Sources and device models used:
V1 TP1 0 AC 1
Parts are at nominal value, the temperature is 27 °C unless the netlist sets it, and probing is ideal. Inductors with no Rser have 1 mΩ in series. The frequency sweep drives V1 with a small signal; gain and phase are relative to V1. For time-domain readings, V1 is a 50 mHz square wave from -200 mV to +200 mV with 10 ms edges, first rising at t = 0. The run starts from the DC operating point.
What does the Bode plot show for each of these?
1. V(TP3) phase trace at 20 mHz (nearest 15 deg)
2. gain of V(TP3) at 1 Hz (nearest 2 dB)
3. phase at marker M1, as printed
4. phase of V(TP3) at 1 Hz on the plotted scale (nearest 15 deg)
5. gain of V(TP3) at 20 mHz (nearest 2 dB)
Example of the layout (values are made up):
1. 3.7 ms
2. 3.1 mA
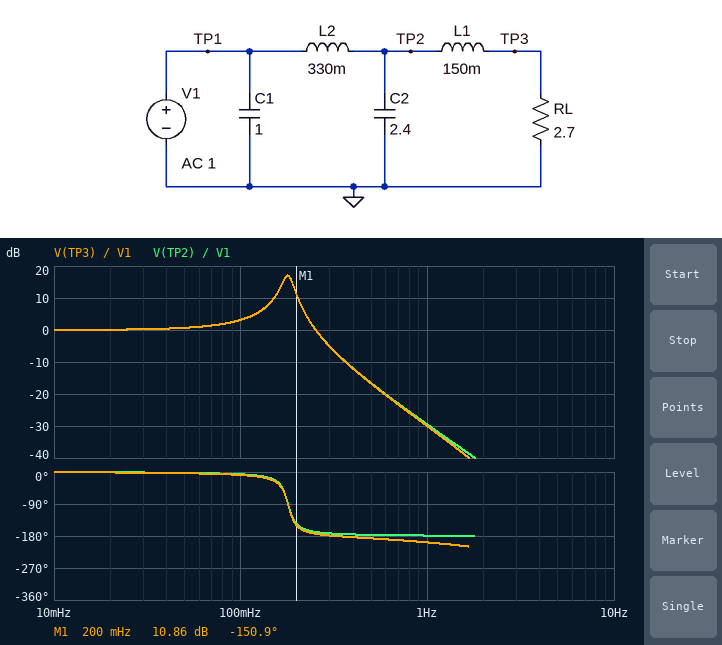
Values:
1. 0 deg
2. -30 dB
3. -150.9 deg
4. -195 deg
5. 0 dB
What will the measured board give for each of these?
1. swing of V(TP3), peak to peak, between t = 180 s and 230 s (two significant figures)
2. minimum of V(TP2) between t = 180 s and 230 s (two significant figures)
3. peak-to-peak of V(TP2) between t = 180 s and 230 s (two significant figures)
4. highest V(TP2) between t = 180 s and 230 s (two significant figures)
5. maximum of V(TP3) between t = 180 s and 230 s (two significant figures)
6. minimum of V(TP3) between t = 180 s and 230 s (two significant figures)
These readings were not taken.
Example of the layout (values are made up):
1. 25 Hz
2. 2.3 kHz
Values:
1. 950 mV
2. -470 mV
3. 950 mV
4. 470 mV
5. 470 mV
6. -470 mV
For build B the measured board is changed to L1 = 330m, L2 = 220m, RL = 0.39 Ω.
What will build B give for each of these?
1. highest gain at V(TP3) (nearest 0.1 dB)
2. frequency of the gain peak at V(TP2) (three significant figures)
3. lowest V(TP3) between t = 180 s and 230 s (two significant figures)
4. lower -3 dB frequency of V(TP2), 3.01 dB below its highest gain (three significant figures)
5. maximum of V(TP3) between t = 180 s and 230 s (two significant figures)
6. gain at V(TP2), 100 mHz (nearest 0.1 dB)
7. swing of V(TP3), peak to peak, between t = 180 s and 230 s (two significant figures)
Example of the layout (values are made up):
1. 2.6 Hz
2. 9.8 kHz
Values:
1. 5.2 dB
2. 264 mHz
3. -270 mV
4. 229 mHz
5. 270 mV
6. 0.2 dB
7. 530 mV
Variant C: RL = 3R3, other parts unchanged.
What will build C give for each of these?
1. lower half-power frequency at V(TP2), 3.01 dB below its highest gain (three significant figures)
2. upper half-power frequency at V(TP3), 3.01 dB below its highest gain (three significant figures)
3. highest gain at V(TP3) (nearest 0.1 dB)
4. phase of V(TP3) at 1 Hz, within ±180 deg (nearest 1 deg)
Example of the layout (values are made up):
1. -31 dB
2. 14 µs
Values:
1. 168 mHz
2. 189 mHz
3. 18.8 dB
4. 165 deg
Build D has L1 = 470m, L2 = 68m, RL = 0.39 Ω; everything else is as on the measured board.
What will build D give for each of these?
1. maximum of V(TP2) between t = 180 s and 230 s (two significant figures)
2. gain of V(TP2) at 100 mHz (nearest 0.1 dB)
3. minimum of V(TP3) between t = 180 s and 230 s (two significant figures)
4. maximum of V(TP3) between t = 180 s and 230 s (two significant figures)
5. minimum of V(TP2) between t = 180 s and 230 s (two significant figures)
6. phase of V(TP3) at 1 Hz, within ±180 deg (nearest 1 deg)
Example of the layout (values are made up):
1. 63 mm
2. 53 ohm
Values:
1. 430 mV
2. 0.1 dB
3. -250 mV
4. 250 mV
5. -430 mV
6. 98 deg
